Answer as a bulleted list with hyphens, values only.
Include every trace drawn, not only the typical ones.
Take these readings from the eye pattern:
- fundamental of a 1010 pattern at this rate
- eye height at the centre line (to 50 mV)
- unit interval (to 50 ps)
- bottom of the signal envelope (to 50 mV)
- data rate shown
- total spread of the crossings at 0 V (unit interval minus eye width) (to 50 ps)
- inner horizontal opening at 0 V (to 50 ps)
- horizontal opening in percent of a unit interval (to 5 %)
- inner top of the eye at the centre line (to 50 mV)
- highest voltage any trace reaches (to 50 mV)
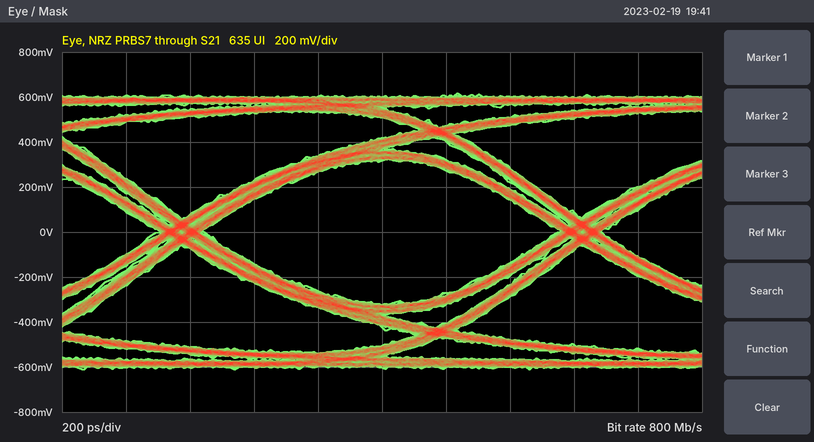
- 400 MHz
- 650 mV
- 1.25 ns
- -600 mV
- 800 Mb/s
- 150 ps
- 1.10 ns
- 90 %
- 300 mV
- 600 mV
